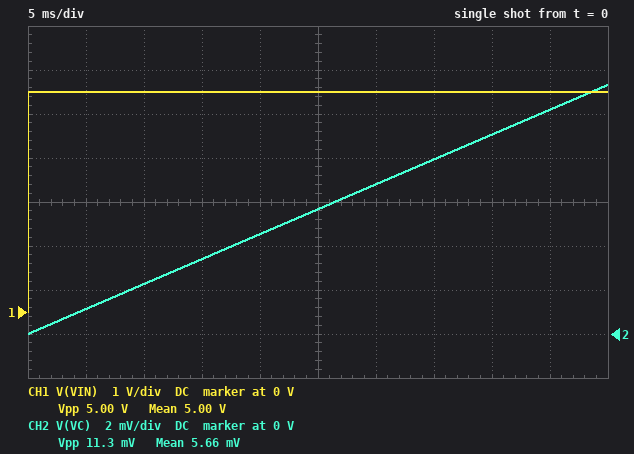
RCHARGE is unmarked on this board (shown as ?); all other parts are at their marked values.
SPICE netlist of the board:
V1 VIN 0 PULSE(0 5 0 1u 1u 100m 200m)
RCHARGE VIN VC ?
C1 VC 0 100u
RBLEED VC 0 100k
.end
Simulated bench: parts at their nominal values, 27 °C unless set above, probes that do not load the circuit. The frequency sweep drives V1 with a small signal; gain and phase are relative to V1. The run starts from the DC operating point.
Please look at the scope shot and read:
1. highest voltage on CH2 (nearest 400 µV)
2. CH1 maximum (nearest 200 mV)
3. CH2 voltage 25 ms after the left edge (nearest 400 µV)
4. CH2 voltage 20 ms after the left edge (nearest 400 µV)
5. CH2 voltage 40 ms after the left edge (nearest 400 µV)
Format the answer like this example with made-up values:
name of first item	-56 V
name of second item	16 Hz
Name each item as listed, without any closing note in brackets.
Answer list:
highest voltage on CH2	11.2 mV
CH1 maximum	5.0 V
CH2 voltage 25 ms after the left edge	5.6 mV
CH2 voltage 20 ms after the left edge	4.4 mV
CH2 voltage 40 ms after the left edge	9.2 mV
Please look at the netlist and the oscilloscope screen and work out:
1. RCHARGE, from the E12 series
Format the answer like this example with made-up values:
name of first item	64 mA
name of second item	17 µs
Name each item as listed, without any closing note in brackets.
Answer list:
RCHARGE, from the E12 series	220 kΩ
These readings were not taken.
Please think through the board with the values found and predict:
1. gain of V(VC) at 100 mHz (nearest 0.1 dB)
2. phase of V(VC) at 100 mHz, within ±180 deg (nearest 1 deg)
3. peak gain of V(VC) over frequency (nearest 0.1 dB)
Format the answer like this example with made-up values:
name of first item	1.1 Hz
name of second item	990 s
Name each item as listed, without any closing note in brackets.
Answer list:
gain of V(VC) at 100 mHz	-23.0 dB
phase of V(VC) at 100 mHz, within ±180 deg	-77 deg
peak gain of V(VC) over frequency	-10.1 dB
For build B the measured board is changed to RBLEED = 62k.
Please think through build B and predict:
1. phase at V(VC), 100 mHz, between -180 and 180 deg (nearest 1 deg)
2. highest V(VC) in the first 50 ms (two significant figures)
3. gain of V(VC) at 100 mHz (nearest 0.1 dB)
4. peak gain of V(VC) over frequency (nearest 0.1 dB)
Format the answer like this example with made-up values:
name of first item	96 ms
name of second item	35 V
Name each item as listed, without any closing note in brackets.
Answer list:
phase at V(VC), 100 mHz, between -180 and 180 deg	-72 deg
highest V(VC) in the first 50 ms	11 mV
gain of V(VC) at 100 mHz	-23.3 dB
peak gain of V(VC) over frequency	-13.2 dB
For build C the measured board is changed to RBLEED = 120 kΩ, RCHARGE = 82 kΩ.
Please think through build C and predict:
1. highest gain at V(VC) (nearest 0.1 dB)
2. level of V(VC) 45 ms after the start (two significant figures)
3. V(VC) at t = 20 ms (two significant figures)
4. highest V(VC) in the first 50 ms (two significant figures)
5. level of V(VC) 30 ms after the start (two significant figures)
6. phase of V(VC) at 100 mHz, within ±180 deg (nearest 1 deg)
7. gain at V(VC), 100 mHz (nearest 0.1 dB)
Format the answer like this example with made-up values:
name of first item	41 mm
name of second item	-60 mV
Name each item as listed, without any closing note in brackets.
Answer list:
highest gain at V(VC)	-4.5 dB
level of V(VC) 45 ms after the start	27 mV
V(VC) at t = 20 ms	12 mV
highest V(VC) in the first 50 ms	30 mV
level of V(VC) 30 ms after the start	18 mV
phase of V(VC) at 100 mHz, within ±180 deg	-72 deg
gain at V(VC), 100 mHz	-14.7 dB
